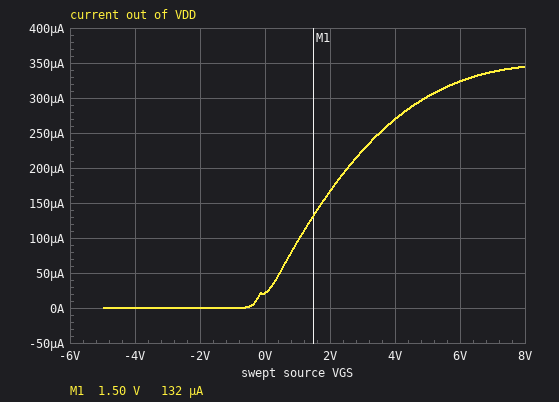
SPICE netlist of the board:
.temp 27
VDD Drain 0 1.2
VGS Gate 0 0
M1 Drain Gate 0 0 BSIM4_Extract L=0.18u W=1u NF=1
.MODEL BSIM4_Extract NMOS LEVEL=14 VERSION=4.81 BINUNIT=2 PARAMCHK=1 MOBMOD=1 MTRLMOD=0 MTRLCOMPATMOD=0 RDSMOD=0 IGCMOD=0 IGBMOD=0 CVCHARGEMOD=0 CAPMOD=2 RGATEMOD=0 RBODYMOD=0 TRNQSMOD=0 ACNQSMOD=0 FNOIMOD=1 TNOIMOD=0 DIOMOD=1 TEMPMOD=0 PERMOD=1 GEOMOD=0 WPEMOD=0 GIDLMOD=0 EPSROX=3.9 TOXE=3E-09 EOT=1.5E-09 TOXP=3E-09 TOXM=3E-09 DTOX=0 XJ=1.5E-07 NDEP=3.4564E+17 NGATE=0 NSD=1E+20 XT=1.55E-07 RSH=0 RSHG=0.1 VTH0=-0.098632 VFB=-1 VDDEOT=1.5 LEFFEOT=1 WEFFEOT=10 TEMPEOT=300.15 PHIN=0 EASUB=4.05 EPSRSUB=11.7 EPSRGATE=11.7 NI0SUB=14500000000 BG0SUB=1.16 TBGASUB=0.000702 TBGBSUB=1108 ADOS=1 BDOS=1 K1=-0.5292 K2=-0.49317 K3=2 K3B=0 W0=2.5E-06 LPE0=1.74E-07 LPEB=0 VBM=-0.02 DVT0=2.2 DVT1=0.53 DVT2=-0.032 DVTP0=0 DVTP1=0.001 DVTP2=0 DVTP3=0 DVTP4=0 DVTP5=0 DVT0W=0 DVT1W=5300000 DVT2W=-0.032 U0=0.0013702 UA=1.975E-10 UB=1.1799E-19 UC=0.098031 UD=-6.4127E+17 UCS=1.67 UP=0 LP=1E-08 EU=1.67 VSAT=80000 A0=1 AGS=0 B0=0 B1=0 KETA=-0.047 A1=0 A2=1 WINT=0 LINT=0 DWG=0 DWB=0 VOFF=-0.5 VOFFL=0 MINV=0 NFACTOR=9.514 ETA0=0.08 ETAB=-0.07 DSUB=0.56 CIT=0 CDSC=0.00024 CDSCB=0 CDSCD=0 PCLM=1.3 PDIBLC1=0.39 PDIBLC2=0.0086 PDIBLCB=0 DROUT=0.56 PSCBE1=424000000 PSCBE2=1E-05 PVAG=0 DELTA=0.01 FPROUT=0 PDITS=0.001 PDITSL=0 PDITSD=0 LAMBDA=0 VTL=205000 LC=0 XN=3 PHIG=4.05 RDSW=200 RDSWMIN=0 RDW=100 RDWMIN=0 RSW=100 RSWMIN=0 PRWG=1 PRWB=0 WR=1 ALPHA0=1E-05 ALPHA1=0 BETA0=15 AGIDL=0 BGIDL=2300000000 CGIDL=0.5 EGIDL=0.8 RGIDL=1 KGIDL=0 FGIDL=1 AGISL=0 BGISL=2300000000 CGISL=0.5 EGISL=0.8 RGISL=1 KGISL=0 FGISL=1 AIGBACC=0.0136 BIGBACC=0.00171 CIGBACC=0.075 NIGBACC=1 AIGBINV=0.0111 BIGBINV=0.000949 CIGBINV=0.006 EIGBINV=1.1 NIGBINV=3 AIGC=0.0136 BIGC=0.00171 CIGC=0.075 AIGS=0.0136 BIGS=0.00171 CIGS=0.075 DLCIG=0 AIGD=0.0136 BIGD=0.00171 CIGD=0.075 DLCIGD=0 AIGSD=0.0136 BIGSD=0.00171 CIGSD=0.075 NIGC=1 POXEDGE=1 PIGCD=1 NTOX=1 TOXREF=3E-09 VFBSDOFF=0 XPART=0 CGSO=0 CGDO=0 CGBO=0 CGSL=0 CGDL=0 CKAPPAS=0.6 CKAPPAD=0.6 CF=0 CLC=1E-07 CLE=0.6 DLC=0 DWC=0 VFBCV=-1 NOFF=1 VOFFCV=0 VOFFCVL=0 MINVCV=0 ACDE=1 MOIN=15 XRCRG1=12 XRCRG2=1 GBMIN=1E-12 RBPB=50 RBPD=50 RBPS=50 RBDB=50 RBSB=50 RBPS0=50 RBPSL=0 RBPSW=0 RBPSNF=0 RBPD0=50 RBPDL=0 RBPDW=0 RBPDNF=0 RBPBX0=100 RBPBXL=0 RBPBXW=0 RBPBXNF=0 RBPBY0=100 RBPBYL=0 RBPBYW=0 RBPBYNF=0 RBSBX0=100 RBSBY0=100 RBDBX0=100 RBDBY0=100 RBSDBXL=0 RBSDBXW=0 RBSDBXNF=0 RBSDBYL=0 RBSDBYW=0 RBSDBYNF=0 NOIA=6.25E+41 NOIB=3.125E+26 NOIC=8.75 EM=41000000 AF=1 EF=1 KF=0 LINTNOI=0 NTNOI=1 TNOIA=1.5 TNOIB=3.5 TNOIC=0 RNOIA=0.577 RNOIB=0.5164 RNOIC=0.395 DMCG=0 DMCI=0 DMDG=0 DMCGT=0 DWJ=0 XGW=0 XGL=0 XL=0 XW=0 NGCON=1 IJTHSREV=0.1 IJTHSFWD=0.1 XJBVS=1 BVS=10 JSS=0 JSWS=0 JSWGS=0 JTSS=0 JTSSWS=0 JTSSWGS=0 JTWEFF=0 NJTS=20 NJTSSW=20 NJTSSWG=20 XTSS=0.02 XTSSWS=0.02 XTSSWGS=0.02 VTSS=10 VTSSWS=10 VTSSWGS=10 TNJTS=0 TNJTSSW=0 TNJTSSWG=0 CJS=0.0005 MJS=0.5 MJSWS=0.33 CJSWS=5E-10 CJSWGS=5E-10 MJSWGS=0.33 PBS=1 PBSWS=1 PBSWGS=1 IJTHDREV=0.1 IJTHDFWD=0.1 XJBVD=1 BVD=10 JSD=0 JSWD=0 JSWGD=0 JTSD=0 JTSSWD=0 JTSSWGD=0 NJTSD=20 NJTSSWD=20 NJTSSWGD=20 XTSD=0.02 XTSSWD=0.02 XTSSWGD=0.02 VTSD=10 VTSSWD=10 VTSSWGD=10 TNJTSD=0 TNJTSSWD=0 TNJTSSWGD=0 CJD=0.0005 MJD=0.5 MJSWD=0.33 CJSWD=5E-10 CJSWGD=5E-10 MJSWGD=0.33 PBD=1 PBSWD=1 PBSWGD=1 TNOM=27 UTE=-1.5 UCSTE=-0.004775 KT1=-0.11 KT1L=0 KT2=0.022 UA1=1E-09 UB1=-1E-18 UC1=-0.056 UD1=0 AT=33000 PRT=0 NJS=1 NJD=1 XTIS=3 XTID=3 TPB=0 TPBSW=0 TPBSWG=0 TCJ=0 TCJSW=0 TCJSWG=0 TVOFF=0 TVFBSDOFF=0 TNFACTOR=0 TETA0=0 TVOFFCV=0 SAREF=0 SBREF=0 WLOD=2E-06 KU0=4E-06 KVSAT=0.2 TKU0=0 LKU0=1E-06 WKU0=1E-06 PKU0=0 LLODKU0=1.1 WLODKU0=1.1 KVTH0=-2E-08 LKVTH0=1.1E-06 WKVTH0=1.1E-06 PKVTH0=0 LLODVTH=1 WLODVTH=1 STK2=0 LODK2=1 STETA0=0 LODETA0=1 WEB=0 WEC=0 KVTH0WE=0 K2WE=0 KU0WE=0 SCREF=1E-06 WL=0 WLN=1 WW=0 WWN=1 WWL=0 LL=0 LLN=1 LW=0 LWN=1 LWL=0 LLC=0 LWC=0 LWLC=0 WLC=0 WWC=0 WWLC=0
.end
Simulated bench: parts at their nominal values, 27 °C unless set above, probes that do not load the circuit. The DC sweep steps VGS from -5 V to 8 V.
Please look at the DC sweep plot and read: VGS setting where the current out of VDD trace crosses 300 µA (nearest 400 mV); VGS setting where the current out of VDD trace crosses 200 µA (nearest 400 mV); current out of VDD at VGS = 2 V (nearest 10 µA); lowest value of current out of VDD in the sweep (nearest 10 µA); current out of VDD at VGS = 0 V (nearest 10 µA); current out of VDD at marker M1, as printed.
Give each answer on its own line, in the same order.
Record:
4.8 V
2.4 V
170 µA
0 A
20 µA
132 µA
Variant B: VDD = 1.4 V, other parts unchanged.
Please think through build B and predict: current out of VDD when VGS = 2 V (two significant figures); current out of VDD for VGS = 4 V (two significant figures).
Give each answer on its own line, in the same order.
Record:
190 µA
310 µA
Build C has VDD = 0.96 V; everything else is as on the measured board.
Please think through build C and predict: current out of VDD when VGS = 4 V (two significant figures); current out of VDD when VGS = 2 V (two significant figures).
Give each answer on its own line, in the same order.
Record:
220 µA
140 µA
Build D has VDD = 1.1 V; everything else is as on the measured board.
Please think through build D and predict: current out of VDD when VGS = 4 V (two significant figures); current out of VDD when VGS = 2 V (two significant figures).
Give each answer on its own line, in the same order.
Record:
250 µA
160 µA
